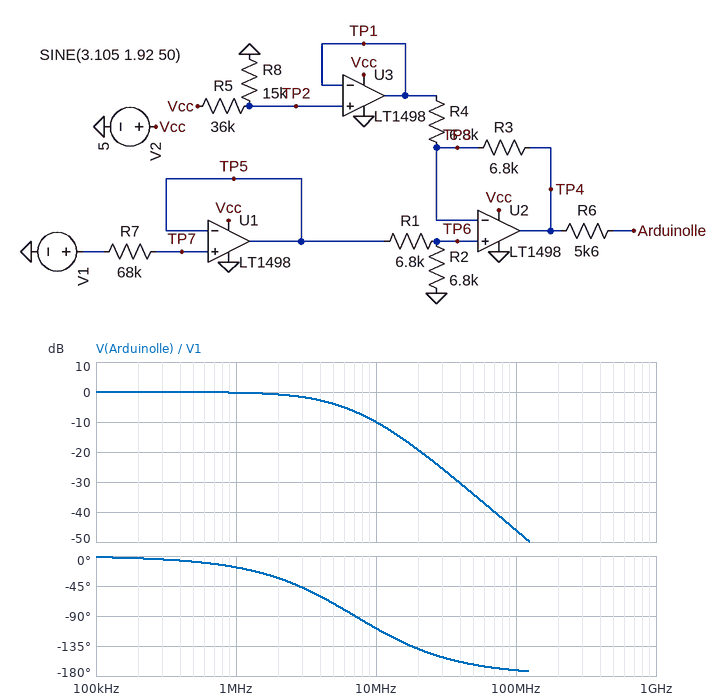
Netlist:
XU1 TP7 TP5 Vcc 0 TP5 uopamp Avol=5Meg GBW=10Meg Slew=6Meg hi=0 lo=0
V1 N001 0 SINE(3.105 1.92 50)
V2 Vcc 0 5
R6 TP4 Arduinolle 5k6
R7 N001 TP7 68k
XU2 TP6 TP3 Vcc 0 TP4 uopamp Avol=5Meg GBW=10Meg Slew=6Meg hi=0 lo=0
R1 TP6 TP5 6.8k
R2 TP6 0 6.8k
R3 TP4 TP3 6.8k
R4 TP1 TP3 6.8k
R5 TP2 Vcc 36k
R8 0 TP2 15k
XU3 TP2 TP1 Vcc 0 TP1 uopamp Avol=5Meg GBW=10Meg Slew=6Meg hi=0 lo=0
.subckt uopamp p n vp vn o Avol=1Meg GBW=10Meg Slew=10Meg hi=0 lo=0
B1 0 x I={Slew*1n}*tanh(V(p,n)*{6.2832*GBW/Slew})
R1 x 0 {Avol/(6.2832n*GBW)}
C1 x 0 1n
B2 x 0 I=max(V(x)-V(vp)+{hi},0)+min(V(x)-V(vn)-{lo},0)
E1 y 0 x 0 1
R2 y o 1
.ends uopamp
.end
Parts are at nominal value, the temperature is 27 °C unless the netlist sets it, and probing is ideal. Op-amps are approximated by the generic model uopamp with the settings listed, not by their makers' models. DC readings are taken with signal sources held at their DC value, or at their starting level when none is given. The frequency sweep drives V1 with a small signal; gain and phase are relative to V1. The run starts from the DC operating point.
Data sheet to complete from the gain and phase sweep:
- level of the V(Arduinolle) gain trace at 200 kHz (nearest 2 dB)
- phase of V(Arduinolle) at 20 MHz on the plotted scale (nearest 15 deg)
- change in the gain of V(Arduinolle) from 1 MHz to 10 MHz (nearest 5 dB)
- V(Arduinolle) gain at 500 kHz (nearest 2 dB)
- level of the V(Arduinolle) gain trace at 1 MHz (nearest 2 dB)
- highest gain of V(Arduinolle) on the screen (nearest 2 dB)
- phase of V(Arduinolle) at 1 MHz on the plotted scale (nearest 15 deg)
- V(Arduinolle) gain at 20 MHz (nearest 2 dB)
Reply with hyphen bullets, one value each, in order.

- 0 dB
- -135 deg
- -10 dB
- 0 dB
- 0 dB
- 0 dB
- -15 deg
- -20 dB
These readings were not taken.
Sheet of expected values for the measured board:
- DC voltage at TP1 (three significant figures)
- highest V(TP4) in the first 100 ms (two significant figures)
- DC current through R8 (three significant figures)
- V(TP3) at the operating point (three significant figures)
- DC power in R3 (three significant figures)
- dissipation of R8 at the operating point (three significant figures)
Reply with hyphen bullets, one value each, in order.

- 1.47 V
- 3.5 V
- 98.0 µA
- 1.55 V
- 987 nW
- 144 µW
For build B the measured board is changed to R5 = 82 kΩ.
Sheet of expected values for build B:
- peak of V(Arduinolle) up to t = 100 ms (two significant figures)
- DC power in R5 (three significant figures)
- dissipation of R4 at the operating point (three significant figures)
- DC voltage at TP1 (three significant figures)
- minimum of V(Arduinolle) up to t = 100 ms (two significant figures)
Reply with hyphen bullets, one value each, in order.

- 4.2 V
- 218 µW
- 89.3 µW
- 773 mV
- 410 mV
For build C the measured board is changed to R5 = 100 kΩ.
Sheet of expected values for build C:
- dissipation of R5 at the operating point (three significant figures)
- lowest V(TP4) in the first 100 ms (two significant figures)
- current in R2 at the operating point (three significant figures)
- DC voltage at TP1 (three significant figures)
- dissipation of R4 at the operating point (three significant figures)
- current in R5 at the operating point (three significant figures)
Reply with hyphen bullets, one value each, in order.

- 189 µW
- 530 mV
- 228 µA
- 652 mV
- 119 µW
- 43.5 µA
